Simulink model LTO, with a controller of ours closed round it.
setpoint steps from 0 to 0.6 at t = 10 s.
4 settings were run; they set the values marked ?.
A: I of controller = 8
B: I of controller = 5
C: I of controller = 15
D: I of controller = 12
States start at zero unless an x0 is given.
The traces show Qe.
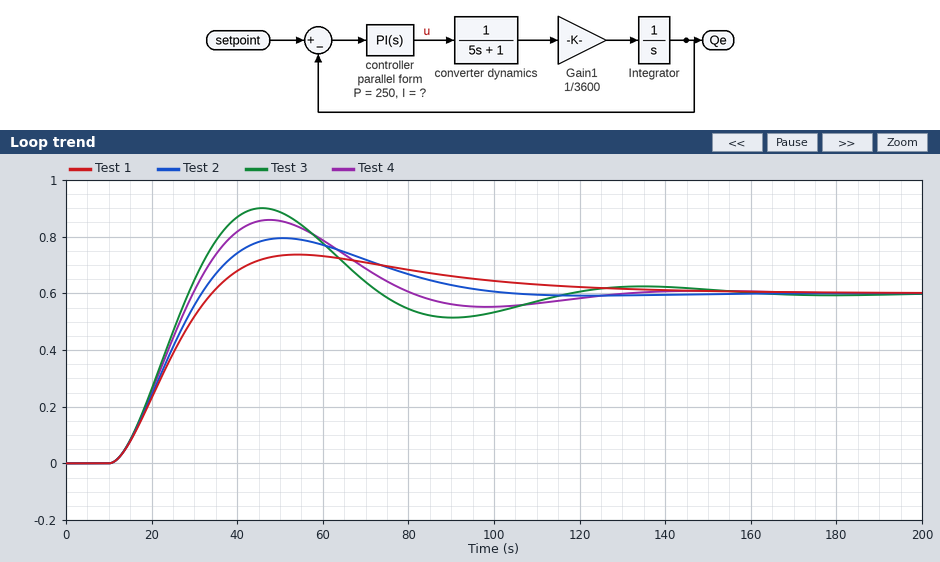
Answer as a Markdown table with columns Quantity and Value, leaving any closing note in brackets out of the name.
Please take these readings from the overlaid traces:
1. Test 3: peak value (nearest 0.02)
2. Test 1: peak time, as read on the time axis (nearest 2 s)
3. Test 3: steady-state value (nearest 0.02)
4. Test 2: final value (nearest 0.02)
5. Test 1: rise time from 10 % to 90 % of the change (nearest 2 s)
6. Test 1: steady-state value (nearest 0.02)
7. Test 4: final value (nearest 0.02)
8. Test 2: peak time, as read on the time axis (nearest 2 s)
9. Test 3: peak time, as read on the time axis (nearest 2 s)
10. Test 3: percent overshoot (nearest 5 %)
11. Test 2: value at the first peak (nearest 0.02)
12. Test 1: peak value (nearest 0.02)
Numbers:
| Quantity | Value |
|---|---|
| Test 3: peak value | 0.90 |
| Test 1: peak time, as read on the time axis | 54 s |
| Test 3: steady-state value | 0.60 |
| Test 2: final value | 0.60 |
| Test 1: rise time from 10 % to 90 % of the change | 16 s |
| Test 1: steady-state value | 0.60 |
| Test 4: final value | 0.60 |
| Test 2: peak time, as read on the time axis | 50 s |
| Test 3: peak time, as read on the time axis | 46 s |
| Test 3: percent overshoot | 50 % |
| Test 2: value at the first peak | 0.80 |
| Test 1: peak value | 0.74 |
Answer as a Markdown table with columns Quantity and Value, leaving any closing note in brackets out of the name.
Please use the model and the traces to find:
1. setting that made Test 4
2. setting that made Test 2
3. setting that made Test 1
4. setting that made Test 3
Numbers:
| Quantity | Value |
|---|---|
| setting that made Test 4 | D |
| setting that made Test 2 | A |
| setting that made Test 1 | B |
| setting that made Test 3 | C |
